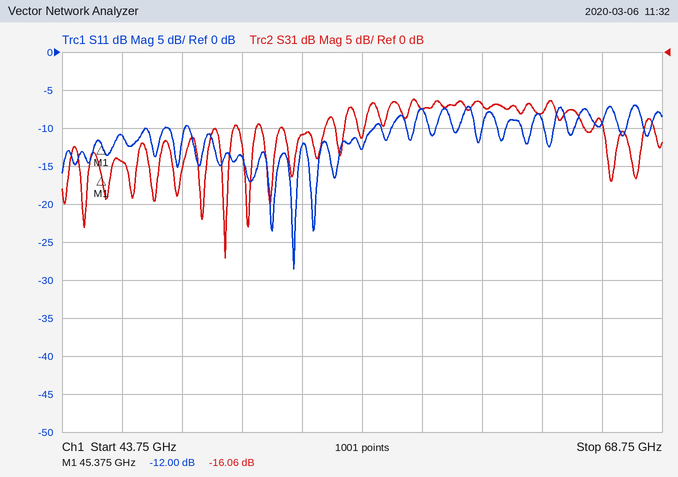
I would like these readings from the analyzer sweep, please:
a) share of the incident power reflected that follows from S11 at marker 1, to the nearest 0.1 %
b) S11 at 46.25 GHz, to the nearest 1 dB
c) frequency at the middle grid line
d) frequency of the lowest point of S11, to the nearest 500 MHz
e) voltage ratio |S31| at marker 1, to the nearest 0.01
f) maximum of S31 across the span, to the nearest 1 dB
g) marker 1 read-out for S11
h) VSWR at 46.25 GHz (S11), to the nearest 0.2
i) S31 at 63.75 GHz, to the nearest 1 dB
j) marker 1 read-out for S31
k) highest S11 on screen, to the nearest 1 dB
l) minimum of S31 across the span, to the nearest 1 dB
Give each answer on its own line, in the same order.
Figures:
6.3 %
-11 dB
56.25 GHz
53.5 GHz
0.16
-6 dB
-12.00 dB
1.8
-8 dB
-16.06 dB
-7 dB
-27 dB
